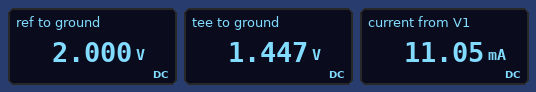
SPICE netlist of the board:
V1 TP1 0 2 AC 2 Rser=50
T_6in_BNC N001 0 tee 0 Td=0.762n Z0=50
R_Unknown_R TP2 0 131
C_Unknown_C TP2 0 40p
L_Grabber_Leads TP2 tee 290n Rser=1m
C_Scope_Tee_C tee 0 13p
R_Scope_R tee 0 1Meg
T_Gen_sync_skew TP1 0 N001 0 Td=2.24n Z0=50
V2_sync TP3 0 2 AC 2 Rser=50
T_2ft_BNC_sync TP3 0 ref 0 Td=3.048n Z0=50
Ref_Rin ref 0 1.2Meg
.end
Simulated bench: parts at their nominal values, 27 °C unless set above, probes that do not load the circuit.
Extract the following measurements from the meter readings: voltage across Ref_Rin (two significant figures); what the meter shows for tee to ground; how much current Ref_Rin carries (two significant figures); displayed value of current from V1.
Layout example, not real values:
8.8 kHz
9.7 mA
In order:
2.0 V
1.447 V
1.7 µA
11.05 mA
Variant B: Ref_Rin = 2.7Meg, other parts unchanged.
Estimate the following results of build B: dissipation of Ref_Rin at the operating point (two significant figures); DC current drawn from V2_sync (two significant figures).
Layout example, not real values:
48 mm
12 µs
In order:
1.5 µW
740 nA
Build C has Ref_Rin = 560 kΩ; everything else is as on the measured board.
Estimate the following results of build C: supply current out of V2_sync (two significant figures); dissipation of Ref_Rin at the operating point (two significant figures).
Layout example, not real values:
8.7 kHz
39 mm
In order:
3.6 µA
7.1 µW
